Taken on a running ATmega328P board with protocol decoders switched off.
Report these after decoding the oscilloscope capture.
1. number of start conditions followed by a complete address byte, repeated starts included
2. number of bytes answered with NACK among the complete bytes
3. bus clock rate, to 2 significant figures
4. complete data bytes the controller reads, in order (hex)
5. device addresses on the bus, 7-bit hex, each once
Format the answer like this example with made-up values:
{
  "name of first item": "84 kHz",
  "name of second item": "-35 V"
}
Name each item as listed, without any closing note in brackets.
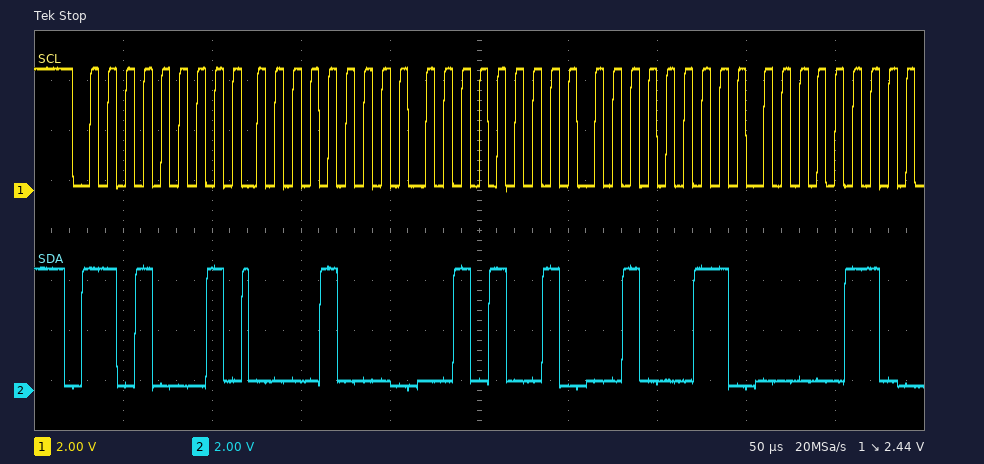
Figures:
{
  "number of start conditions followed by a complete address byte, repeated starts included": "1",
  "number of bytes answered with NACK among the complete bytes": "0",
  "bus clock rate, to 2 significant figures": "100 kHz",
  "complete data bytes the controller reads, in order": "08 29 23 06",
  "device addresses on the bus, 7-bit hex, each once": "0x68"
}
